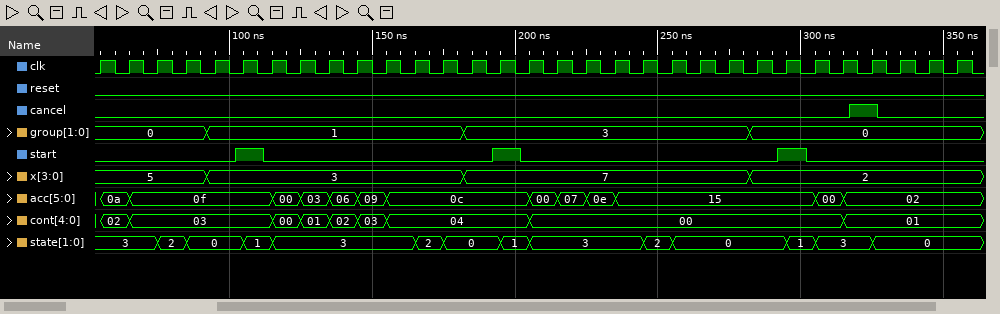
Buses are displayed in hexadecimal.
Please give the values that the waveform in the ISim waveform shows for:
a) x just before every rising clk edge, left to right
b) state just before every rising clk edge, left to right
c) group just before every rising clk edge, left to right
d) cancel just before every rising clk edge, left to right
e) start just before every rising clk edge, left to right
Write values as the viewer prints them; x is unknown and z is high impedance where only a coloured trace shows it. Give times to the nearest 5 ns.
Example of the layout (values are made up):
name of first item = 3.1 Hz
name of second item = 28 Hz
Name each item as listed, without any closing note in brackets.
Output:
x just before every rising clk edge, left to right = 5, 5, 5, 5, 3, 3, 3, 3, 3, 3, 3, 3, 3, 7, 7, 7, 7, 7, 7, 7, 7, 7, 7, 2, 2, 2, 2, 2, 2, 2, 2
state just before every rising clk edge, left to right = 3, 3, 3, 2, 0, 0, 1, 3, 3, 3, 3, 3, 2, 0, 0, 1, 3, 3, 3, 3, 2, 0, 0, 0, 0, 1, 3, 3, 0, 0, 0
group just before every rising clk edge, left to right = 0, 0, 0, 0, 1, 1, 1, 1, 1, 1, 1, 1, 1, 3, 3, 3, 3, 3, 3, 3, 3, 3, 3, 0, 0, 0, 0, 0, 0, 0, 0
cancel just before every rising clk edge, left to right = 0 0 0 0 0 0 0 0 0 0 0 0 0 0 0 0 0 0 0 0 0 0 0 0 0 0 0 1 0 0 0
start just before every rising clk edge, left to right = 0 0 0 0 0 1 0 0 0 0 0 0 0 0 1 0 0 0 0 0 0 0 0 0 1 0 0 0 0 0 0
